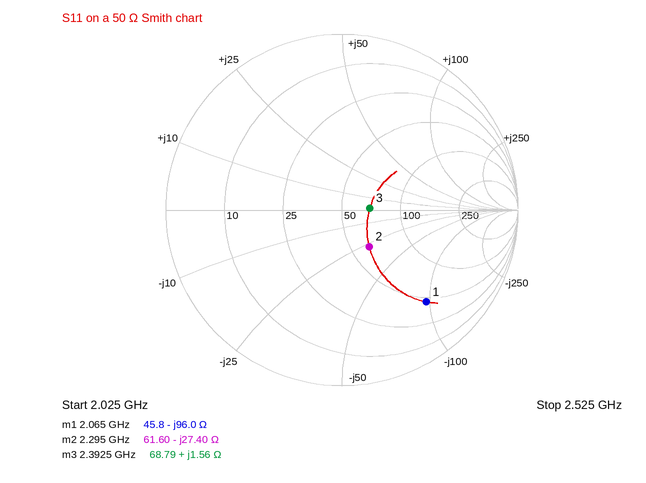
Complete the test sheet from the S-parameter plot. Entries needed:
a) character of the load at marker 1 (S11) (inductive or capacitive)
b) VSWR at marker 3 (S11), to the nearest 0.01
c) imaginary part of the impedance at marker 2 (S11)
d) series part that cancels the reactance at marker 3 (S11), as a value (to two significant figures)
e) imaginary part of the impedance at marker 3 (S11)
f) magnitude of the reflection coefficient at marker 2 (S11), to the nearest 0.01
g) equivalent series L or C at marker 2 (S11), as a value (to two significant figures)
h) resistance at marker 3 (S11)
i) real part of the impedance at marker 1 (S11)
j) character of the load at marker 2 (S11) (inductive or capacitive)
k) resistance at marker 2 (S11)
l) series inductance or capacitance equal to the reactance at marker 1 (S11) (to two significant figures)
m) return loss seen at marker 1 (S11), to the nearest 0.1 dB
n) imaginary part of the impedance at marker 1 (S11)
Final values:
capacitive
1.38
-27.40 Ω
43 pF
+1.56 Ω
0.26
2.5 pF
68.79 Ω
45.8 Ω
capacitive
61.60 Ω
800 fF
3.0 dB
-96.0 Ω
